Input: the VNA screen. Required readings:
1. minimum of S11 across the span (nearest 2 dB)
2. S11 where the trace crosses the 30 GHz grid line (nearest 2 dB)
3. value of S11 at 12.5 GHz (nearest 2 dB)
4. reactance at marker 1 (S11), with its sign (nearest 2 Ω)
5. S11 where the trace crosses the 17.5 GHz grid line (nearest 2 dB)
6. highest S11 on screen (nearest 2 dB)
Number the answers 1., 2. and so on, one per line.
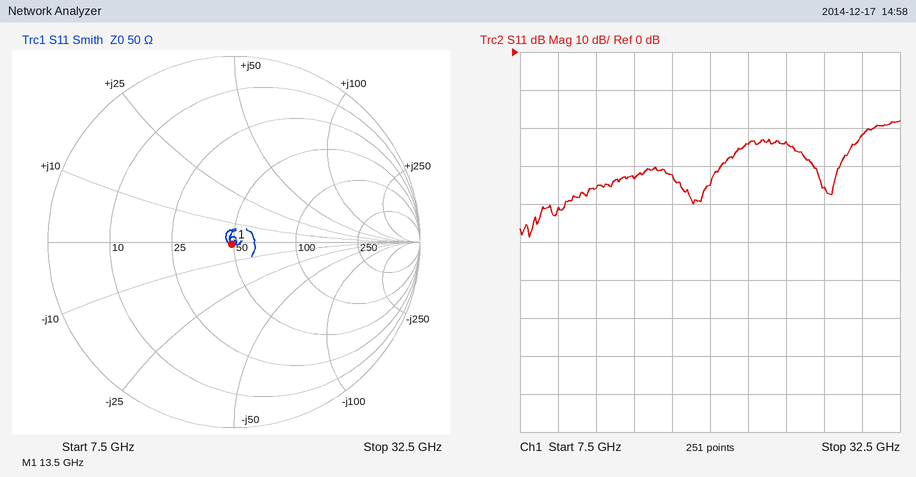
1. -48 dB
2. -22 dB
3. -36 dB
4. -2 Ω
5. -32 dB
6. -18 dB
